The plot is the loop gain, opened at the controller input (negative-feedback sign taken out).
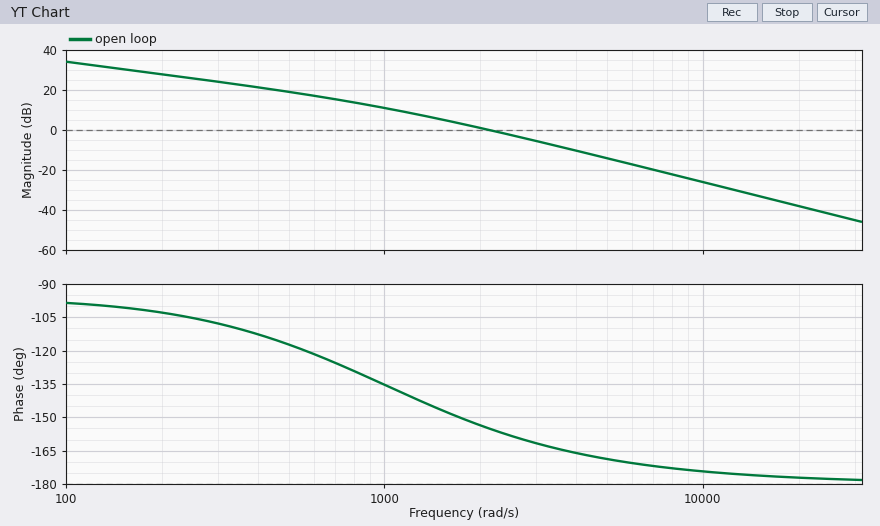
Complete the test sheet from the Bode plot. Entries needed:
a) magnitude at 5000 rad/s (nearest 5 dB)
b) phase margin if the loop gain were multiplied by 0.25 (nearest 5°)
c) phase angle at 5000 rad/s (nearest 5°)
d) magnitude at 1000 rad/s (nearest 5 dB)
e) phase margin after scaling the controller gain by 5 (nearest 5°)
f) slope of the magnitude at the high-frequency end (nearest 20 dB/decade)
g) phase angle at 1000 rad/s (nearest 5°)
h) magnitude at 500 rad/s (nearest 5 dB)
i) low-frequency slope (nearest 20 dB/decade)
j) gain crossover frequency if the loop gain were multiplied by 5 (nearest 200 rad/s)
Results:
-15 dB
45°
-170°
10 dB
10°
-40 dB/decade
-135°
20 dB
-20 dB/decade
5000 rad/s
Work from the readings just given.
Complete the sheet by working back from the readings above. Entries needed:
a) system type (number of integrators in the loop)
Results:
1
